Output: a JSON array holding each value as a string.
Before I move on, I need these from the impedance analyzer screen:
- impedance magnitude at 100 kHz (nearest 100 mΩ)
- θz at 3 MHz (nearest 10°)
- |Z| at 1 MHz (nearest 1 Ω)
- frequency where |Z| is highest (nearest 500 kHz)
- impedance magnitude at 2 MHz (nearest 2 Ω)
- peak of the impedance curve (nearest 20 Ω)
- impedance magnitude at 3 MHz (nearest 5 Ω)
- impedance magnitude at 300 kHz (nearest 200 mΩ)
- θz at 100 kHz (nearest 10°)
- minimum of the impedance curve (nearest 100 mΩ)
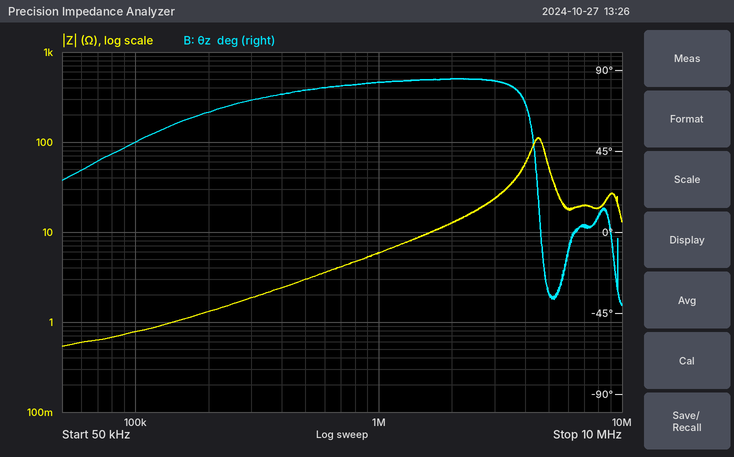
["800 mΩ", "80°", "6 Ω", "4.5 MHz", "12 Ω", "120 Ω", "25 Ω", "1.8 Ω", "50°", "500 mΩ"]
